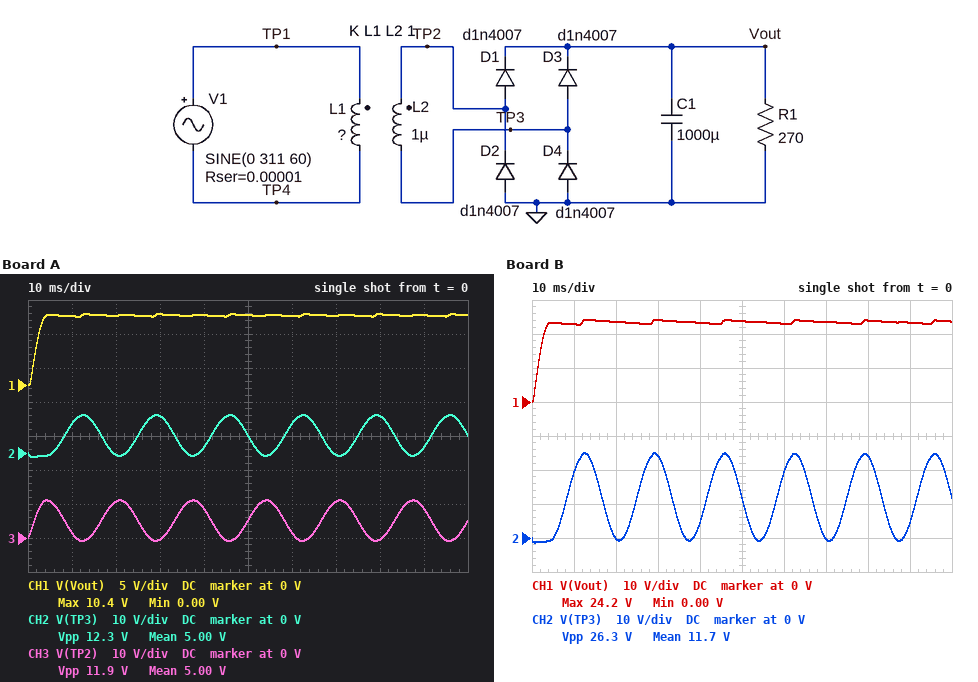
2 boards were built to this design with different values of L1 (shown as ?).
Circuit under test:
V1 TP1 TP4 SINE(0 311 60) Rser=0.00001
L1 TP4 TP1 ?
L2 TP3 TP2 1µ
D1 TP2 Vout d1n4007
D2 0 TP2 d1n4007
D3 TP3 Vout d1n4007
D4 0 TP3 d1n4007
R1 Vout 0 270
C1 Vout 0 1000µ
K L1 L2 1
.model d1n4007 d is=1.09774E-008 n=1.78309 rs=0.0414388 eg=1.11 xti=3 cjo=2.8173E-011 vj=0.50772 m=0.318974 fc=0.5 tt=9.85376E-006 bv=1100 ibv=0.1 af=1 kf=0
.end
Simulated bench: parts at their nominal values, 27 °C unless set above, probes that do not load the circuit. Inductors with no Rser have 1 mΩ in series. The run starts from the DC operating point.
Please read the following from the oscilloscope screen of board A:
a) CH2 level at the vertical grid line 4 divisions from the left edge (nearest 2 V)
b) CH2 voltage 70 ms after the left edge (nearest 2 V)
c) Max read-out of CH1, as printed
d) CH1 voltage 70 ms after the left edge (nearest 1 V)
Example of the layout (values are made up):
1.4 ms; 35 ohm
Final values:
2 V; 0 V; 10.4 V; 10 V
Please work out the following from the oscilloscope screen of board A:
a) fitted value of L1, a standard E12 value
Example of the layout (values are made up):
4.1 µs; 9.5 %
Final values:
680 µH
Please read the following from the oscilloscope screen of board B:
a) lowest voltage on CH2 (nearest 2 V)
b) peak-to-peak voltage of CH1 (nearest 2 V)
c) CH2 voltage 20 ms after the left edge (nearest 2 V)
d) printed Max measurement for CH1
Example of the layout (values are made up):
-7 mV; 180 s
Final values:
-2 V; 24 V; 0 V; 24.2 V
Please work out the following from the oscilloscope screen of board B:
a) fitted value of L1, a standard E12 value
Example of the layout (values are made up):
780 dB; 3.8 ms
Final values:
150 µH
